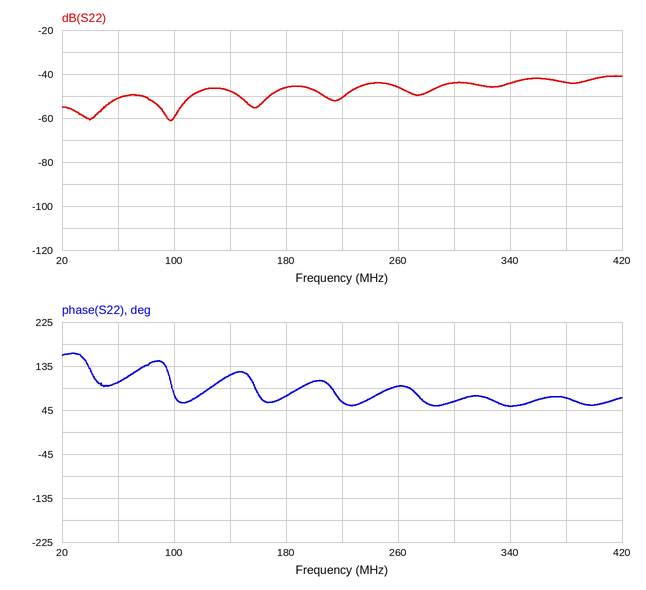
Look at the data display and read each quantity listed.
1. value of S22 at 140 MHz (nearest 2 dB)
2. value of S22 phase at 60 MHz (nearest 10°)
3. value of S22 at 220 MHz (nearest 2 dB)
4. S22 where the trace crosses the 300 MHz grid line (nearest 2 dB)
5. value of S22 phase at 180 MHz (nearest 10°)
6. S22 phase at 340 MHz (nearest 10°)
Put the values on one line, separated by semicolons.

-48 dB; 100°; -50 dB; -44 dB; 70°; 50°
